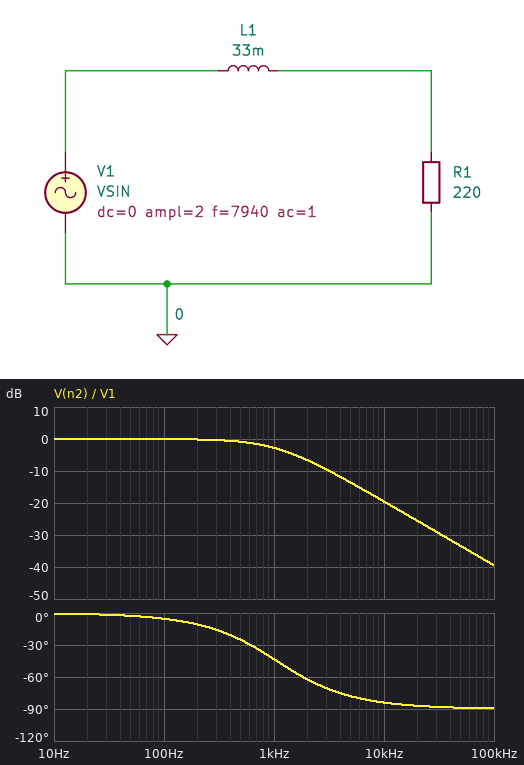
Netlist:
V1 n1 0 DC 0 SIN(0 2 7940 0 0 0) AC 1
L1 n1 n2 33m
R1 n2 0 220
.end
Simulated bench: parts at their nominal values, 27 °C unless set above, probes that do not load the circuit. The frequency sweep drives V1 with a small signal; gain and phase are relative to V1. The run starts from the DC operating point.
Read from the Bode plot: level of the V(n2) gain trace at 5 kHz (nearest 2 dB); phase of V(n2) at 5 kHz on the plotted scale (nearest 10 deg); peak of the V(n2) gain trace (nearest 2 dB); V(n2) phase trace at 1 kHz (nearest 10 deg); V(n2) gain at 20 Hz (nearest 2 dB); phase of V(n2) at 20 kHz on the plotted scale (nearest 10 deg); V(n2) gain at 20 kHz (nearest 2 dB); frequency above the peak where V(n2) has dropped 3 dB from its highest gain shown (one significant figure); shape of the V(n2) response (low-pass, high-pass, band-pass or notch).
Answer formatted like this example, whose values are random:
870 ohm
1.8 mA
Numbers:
-14 dB
-80 deg
0 dB
-40 deg
0 dB
-90 deg
-26 dB
1 kHz
low-pass
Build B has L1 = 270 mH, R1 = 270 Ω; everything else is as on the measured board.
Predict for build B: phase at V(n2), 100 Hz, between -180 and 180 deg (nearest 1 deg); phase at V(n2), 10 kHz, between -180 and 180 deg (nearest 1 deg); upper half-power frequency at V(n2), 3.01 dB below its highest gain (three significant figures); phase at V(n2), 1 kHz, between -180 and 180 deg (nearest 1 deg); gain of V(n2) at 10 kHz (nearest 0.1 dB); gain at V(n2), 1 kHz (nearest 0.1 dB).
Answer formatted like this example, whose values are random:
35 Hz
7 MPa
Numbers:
-32 deg
-89 deg
159 Hz
-81 deg
-36.0 dB
-16.1 dB
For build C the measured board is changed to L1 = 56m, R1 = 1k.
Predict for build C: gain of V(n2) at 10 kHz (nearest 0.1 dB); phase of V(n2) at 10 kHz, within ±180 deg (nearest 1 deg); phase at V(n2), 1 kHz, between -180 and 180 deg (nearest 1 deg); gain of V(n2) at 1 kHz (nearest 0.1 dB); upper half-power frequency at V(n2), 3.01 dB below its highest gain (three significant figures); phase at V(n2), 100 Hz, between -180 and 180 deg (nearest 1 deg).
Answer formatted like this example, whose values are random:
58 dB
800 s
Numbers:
-11.3 dB
-74 deg
-19 deg
-0.5 dB
2.84 kHz
-2 deg
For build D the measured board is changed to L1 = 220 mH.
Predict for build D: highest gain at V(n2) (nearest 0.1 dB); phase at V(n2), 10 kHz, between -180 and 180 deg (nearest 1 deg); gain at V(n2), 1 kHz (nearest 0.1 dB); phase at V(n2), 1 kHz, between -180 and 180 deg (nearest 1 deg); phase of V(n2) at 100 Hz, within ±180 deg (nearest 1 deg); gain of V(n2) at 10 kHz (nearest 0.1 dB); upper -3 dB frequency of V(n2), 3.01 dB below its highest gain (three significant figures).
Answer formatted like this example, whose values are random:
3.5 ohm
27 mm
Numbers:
0 dB
-89 deg
-16.1 dB
-81 deg
-32 deg
-36.0 dB
159 Hz
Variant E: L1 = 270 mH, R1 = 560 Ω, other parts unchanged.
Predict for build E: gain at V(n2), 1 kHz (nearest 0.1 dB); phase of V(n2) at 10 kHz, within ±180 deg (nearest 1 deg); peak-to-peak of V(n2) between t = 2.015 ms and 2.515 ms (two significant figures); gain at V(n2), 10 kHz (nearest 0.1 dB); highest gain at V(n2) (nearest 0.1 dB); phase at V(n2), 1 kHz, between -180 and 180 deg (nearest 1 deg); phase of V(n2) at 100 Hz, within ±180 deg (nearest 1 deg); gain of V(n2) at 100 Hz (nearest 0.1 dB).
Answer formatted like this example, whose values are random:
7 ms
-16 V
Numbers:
-10.1 dB
-88 deg
170 mV
-29.6 dB
0 dB
-72 deg
-17 deg
-0.4 dB
